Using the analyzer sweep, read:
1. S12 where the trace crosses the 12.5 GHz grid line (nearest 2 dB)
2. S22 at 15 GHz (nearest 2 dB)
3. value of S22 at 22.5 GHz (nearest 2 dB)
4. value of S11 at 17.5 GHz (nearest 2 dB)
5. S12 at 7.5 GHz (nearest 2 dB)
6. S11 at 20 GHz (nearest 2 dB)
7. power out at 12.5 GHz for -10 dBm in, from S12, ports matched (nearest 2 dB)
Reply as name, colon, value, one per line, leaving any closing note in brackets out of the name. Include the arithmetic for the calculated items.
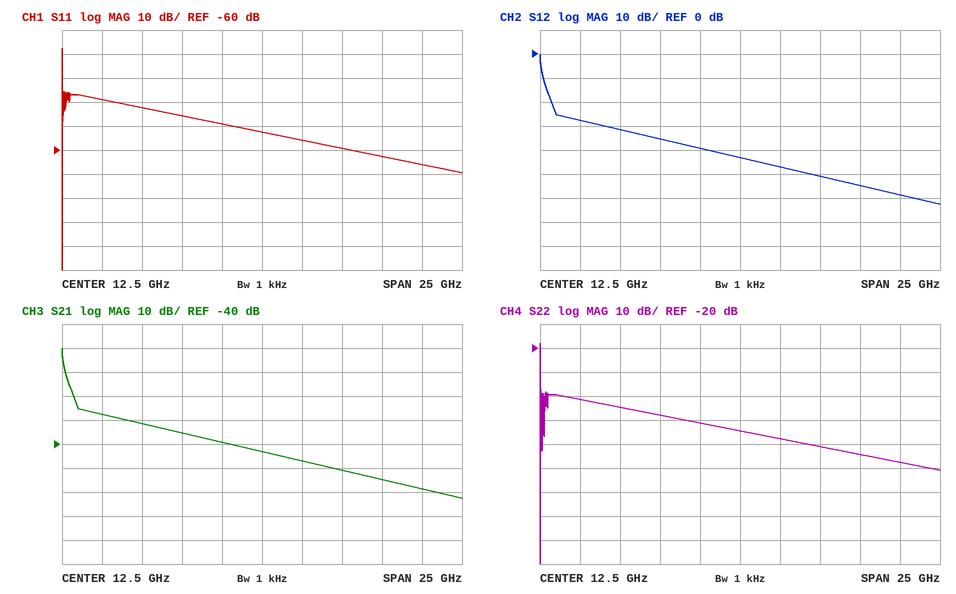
S12 where the trace crosses the 12.5 GHz grid line: -44 dB
S22 at 15 GHz: -58 dB
value of S22 at 22.5 GHz: -68 dB
value of S11 at 17.5 GHz: -60 dB
S12 at 7.5 GHz: -36 dB
S11 at 20 GHz: -62 dB
power out at 12.5 GHz for -10 dBm in, from S12, ports matched: -10 dBm + (-44 dB) = -54 dBm
